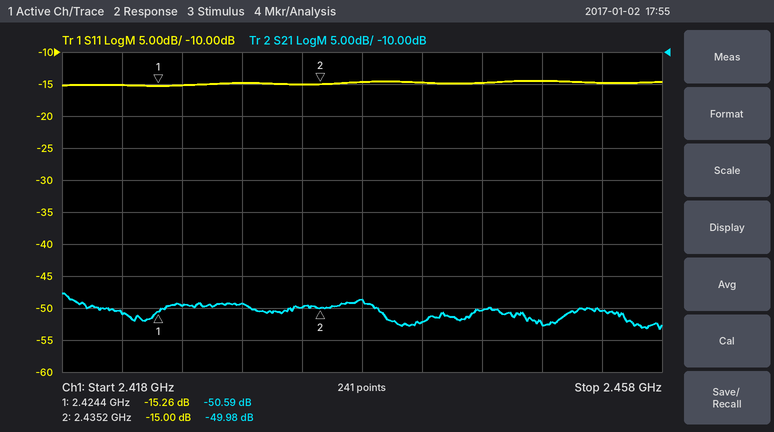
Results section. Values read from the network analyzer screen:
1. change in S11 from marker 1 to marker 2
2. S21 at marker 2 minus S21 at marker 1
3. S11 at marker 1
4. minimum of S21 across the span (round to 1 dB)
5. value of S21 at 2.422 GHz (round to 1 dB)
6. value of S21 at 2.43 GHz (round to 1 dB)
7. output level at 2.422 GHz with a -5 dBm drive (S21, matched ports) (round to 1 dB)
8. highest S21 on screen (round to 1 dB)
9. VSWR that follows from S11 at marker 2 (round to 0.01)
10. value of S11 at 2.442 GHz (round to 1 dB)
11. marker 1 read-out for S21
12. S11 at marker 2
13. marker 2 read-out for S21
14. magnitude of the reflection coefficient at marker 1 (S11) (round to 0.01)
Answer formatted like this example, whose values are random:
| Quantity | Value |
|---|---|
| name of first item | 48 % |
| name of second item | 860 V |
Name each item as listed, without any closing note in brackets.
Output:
| Quantity | Value |
|---|---|
| change in S11 from marker 1 to marker 2 | 0.26 dB |
| S21 at marker 2 minus S21 at marker 1 | 0.61 dB |
| S11 at marker 1 | -15.26 dB |
| minimum of S21 across the span | -53 dB |
| value of S21 at 2.422 GHz | -51 dB |
| value of S21 at 2.43 GHz | -49 dB |
| output level at 2.422 GHz with a -5 dBm drive (S21, matched ports) | -56 dBm |
| highest S21 on screen | -48 dB |
| VSWR that follows from S11 at marker 2 | 1.43 |
| value of S11 at 2.442 GHz | -15 dB |
| marker 1 read-out for S21 | -50.59 dB |
| S11 at marker 2 | -15.00 dB |
| marker 2 read-out for S21 | -49.98 dB |
| magnitude of the reflection coefficient at marker 1 (S11) | 0.17 |
